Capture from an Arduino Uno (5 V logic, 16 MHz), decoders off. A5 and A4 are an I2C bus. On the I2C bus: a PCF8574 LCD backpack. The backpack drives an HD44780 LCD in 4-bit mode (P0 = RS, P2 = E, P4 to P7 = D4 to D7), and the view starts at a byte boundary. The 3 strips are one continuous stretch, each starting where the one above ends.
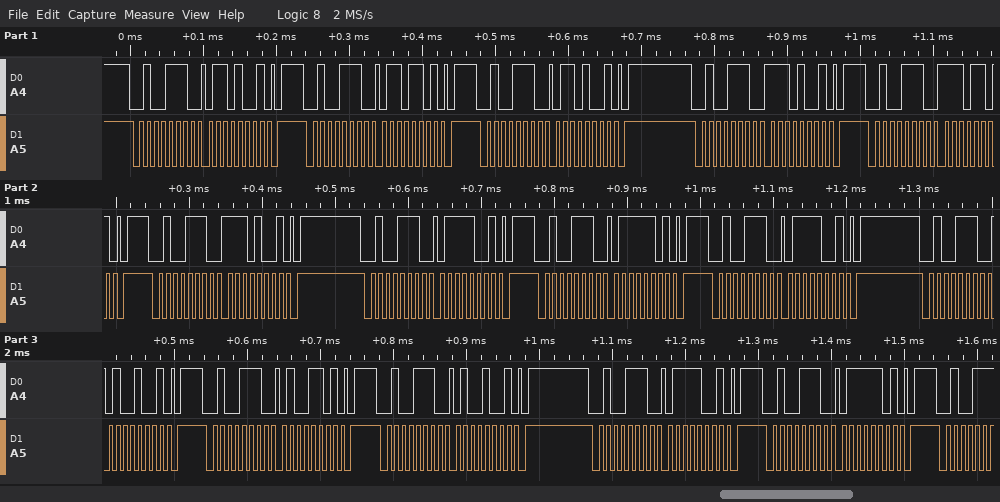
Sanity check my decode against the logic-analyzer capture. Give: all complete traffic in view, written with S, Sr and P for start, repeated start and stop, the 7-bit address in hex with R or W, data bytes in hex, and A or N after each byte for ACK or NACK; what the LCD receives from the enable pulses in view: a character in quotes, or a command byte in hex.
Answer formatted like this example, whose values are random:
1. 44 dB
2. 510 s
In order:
1. S 27W A 69 A P S 27W A 6D A P S 27W A 69 A P S 27W A E9 A P S 27W A ED A P S 27W A E9 A P S 27W A 79 A P S 27W A 7D A P S 27W A 79 A P S 27W A 49 A P S 27W A 4D A P S 27W A 49 A P S 27W A 79 A P S 27W A 7D A P
2. 'n' 't'
